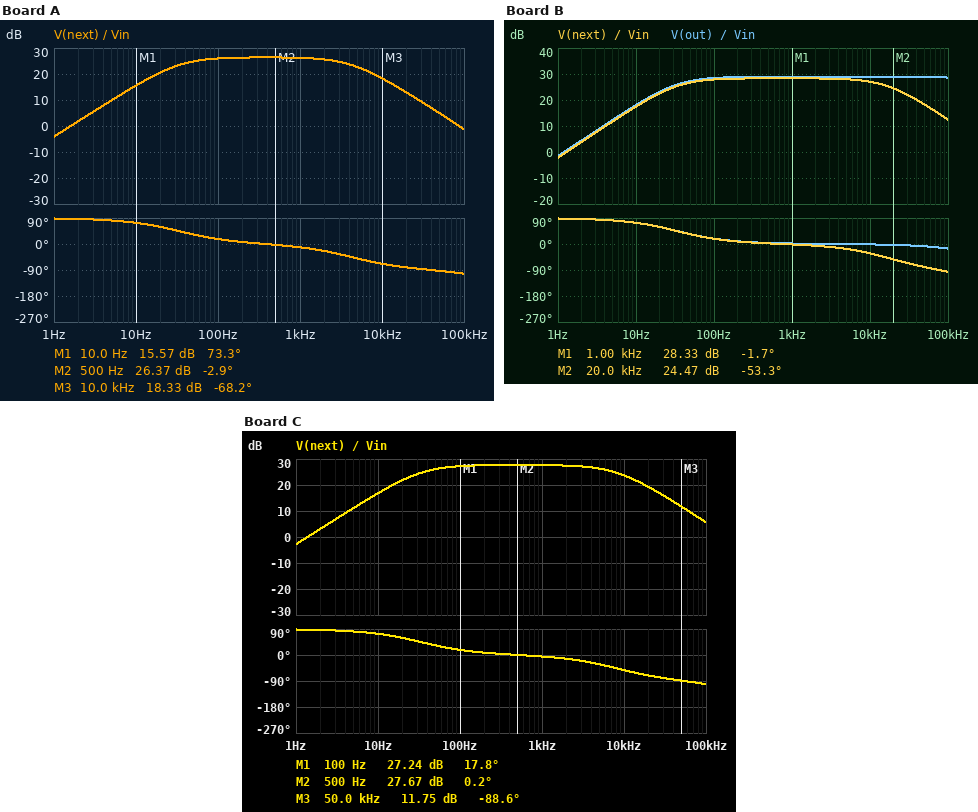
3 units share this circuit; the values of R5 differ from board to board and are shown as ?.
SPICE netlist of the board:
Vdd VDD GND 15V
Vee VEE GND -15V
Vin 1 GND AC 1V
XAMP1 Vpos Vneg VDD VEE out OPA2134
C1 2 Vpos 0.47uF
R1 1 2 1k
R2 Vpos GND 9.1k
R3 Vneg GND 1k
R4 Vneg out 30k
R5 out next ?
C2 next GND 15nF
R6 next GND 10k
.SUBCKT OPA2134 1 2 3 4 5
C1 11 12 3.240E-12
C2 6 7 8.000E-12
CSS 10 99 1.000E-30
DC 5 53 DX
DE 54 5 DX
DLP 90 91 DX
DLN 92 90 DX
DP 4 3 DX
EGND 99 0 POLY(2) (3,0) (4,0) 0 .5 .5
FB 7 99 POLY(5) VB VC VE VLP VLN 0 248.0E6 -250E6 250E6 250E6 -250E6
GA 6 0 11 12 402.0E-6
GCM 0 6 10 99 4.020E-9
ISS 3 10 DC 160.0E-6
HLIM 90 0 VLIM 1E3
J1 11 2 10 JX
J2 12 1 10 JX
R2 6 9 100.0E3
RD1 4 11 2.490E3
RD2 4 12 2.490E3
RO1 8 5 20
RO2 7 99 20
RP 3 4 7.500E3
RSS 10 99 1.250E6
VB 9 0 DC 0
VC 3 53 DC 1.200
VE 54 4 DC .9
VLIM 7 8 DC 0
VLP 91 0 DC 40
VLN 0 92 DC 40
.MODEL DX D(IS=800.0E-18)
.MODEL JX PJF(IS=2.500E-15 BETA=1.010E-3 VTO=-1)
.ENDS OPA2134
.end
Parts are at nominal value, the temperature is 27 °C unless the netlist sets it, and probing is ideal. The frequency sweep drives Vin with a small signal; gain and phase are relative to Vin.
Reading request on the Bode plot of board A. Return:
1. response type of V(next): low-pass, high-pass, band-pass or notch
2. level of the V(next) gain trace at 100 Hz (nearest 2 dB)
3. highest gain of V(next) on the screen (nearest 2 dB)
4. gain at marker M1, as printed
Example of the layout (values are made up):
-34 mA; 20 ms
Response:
band-pass; 26 dB; 26 dB; 15.57 dB
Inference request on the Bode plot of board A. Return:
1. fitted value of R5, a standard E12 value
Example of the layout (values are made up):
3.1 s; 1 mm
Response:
3.3 kΩ
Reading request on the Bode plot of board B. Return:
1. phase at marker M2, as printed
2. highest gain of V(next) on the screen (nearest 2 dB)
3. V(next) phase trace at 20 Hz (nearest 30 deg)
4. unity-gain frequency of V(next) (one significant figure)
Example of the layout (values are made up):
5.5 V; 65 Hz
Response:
-53.3 deg; 28 dB; 60 deg; 1 Hz
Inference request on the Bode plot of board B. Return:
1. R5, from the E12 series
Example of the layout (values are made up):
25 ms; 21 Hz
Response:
680 Ω
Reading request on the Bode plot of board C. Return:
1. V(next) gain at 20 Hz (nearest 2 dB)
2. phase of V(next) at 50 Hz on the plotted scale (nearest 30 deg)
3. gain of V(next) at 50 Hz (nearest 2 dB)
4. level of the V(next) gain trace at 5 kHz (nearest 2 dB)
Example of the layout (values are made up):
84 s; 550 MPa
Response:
22 dB; 30 deg; 26 dB; 26 dB
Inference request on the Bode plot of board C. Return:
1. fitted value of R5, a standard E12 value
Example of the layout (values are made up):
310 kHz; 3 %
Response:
1.5 kΩ
